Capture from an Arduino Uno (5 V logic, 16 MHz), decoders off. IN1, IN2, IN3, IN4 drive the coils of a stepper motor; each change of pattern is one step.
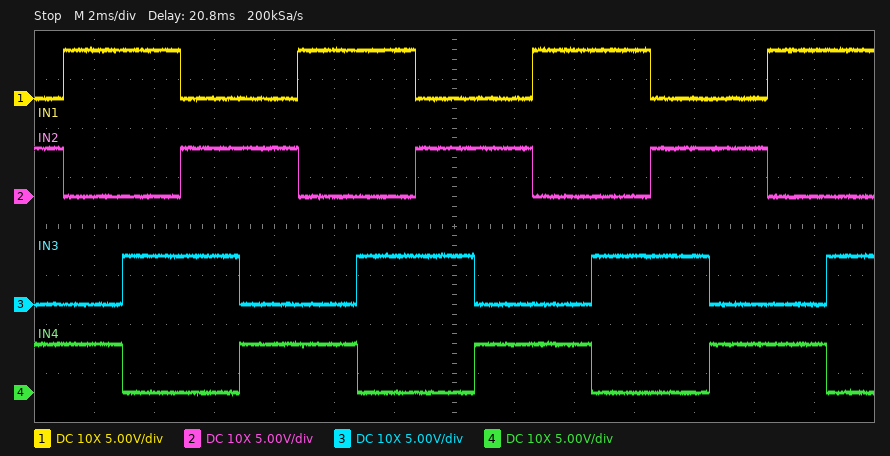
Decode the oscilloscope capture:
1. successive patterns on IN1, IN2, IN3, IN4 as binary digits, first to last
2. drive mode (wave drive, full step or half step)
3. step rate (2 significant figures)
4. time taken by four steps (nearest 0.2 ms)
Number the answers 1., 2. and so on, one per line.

1. 0101 1001 1010 0110 0101 1001 1010 0110 0101 1001 1010 0110 0101 1001 1010
2. full step
3. 510 steps/s
4. 7.8 ms
